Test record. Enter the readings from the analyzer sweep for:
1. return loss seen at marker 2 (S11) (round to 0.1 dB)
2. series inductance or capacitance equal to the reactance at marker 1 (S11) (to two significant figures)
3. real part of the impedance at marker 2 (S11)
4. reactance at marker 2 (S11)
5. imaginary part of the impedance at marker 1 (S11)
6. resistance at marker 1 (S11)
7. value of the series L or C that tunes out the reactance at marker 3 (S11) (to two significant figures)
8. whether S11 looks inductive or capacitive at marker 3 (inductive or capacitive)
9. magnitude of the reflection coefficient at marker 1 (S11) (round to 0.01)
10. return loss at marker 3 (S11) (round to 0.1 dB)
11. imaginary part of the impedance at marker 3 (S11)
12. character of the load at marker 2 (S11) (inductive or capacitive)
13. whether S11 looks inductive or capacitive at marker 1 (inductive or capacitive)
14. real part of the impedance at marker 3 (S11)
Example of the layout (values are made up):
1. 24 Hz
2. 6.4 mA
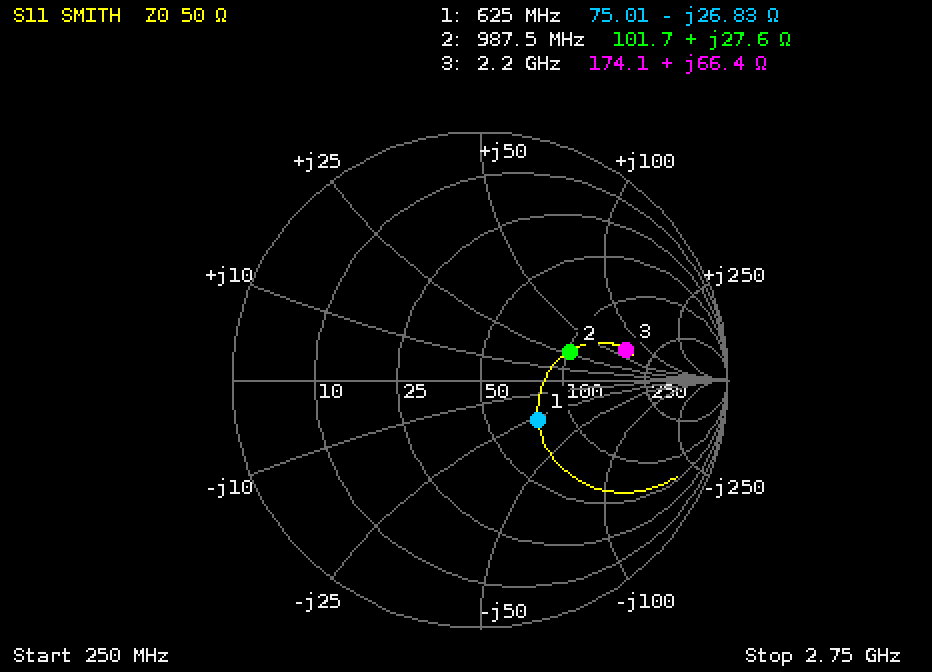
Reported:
1. 8.4 dB
2. 9.5 pF
3. 101.7 Ω
4. +27.6 Ω
5. -26.83 Ω
6. 75.01 Ω
7. 1.1 pF
8. inductive
9. 0.29
10. 4.4 dB
11. +66.4 Ω
12. inductive
13. capacitive
14. 174.1 Ω
